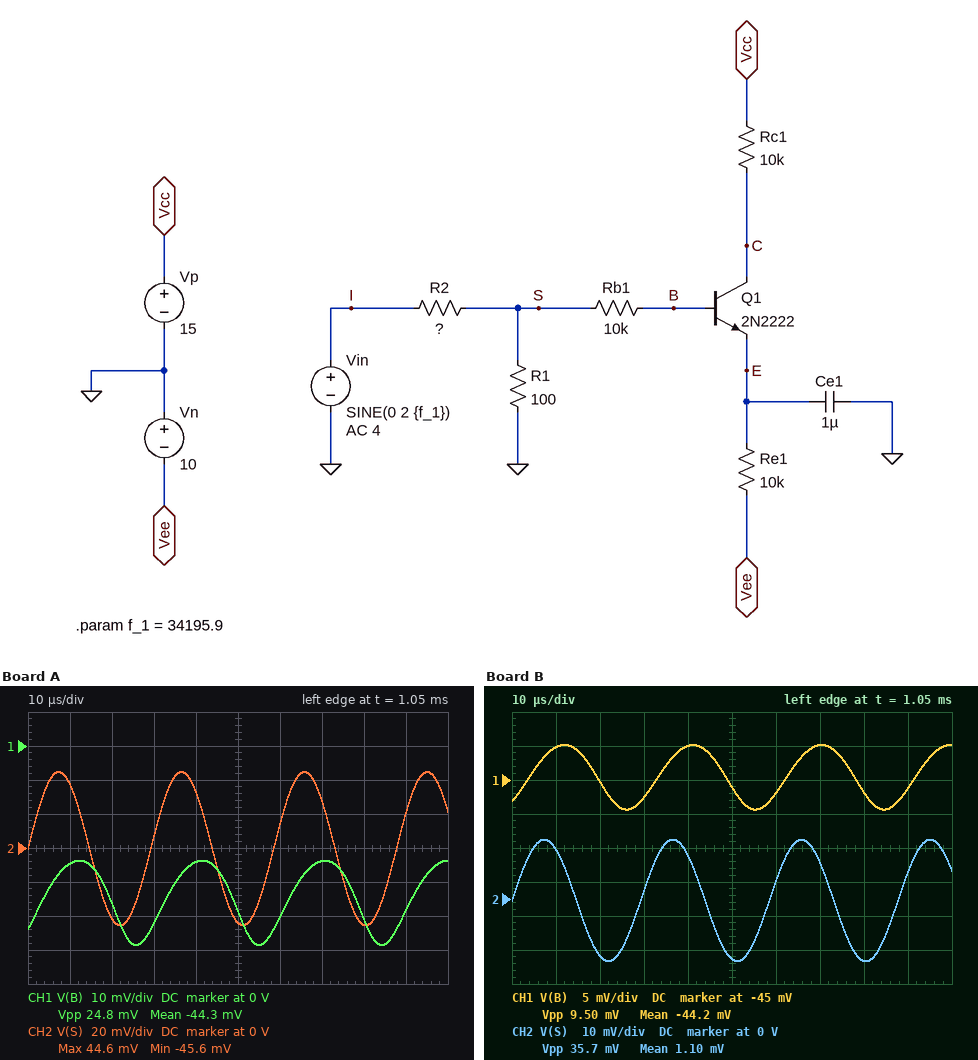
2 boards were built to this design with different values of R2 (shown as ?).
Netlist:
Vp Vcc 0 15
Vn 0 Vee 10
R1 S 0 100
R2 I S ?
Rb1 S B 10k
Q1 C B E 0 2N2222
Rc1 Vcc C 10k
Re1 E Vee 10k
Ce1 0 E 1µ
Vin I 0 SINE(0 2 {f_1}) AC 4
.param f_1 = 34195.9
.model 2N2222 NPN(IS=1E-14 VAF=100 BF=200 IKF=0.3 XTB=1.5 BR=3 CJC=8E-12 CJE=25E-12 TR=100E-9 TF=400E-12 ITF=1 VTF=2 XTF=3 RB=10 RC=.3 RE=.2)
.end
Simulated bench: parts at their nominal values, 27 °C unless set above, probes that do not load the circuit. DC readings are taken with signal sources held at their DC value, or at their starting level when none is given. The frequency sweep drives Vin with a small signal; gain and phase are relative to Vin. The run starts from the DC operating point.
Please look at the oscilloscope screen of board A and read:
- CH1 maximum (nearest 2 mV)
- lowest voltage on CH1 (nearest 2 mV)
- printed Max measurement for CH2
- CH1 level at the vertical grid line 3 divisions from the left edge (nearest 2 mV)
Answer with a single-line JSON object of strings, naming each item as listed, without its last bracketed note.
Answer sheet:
{"CH1 maximum": "-34 mV", "lowest voltage on CH1": "-58 mV", "printed Max measurement for CH2": "44.6 mV", "CH1 level at the vertical grid line 3 divisions from the left edge": "-52 mV"}
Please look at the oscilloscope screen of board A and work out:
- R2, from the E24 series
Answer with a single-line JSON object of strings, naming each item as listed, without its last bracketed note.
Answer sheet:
{"R2, from the E24 series": "4.3 kΩ"}
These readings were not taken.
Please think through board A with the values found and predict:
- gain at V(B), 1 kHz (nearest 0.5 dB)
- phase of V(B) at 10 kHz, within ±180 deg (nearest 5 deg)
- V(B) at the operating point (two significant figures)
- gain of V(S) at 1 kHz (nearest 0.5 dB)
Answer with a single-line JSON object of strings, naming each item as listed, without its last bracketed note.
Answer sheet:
{"gain at V(B), 1 kHz": "-33.5 dB", "phase of V(B) at 10 kHz, within ±180 deg": "-35 deg", "V(B) at the operating point": "-44 mV", "gain of V(S) at 1 kHz": "-33.0 dB"}
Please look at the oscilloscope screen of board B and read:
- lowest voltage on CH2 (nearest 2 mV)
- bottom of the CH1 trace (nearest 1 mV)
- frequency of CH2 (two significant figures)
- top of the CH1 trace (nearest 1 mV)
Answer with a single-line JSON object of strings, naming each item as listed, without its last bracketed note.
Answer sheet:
{"lowest voltage on CH2": "-18 mV", "bottom of the CH1 trace": "-49 mV", "frequency of CH2": "34 kHz", "top of the CH1 trace": "-40 mV"}
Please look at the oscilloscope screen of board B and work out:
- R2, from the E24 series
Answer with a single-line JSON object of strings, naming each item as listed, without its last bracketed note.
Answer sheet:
{"R2, from the E24 series": "11 kΩ"}
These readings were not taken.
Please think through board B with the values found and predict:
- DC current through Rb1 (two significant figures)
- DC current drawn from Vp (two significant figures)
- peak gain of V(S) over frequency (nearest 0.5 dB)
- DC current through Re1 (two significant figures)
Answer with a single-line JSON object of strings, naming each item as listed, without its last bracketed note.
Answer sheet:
{"DC current through Rb1": "4.4 µA", "DC current drawn from Vp": "930 µA", "peak gain of V(S) over frequency": "-41.0 dB", "DC current through Re1": "930 µA"}
